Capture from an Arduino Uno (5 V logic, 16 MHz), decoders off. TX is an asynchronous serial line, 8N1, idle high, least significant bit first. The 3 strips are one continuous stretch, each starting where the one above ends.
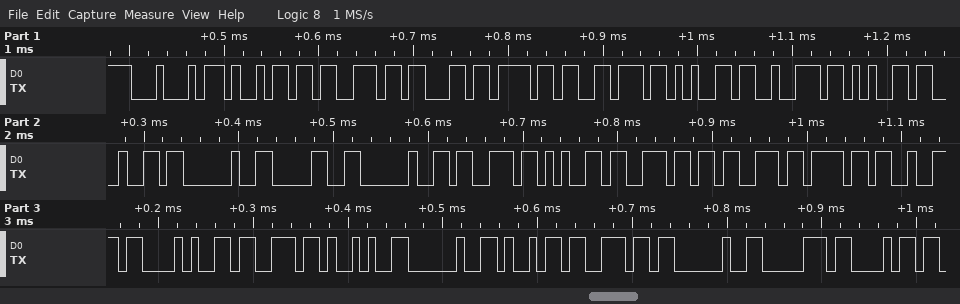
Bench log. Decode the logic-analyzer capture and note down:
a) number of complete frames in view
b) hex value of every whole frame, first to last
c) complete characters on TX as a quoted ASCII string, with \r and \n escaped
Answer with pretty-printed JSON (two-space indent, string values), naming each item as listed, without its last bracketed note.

{
  "number of complete frames in view": "28",
  "hex value of every whole frame, first to last": "44 69 73 63 6F 76 65 72 65 64 20 30 20 73 65 6E 73 6F 72 28 73 29 20 69 6E 20 70 68",
  "complete characters on TX as a quoted ASCII string, with \\r and \\n escaped": "\"Discovered 0 sensor(s) in ph\""
}
